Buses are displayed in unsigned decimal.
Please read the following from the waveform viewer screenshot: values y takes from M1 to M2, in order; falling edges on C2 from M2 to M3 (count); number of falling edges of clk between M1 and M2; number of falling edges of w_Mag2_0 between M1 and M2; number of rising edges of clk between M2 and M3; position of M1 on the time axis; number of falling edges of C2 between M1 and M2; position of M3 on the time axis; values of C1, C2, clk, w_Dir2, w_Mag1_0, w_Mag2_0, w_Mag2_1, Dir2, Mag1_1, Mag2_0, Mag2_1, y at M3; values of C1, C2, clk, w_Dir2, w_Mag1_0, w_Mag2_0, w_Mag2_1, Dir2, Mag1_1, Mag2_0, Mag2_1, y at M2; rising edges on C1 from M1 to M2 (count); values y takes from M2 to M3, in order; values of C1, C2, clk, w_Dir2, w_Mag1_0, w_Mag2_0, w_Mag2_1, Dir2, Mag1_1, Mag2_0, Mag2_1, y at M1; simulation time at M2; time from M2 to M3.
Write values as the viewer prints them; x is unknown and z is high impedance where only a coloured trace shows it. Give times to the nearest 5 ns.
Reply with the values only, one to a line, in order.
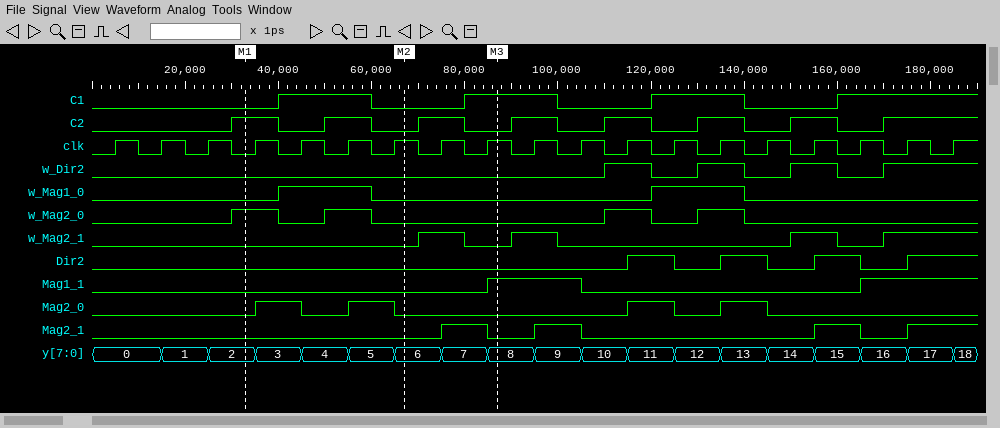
2, 3, 4, 5, 6
1
3
2
2
35 ns
2
85 ns
C1=1, C2=0, clk=1, w_Dir2=0, w_Mag1_0=0, w_Mag2_0=0, w_Mag2_1=0, Dir2=0, Mag1_1=1, Mag2_0=0, Mag2_1=0, y=8
C1=0, C2=0, clk=1, w_Dir2=0, w_Mag1_0=0, w_Mag2_0=0, w_Mag2_1=0, Dir2=0, Mag1_1=0, Mag2_0=0, Mag2_1=0, y=6
1
6, 7, 8
C1=0, C2=1, clk=0, w_Dir2=0, w_Mag1_0=0, w_Mag2_0=1, w_Mag2_1=0, Dir2=0, Mag1_1=0, Mag2_0=0, Mag2_1=0, y=2
65 ns
20 ns
